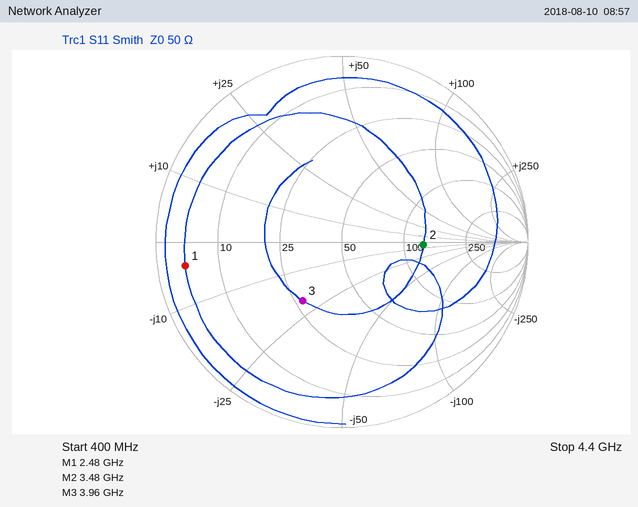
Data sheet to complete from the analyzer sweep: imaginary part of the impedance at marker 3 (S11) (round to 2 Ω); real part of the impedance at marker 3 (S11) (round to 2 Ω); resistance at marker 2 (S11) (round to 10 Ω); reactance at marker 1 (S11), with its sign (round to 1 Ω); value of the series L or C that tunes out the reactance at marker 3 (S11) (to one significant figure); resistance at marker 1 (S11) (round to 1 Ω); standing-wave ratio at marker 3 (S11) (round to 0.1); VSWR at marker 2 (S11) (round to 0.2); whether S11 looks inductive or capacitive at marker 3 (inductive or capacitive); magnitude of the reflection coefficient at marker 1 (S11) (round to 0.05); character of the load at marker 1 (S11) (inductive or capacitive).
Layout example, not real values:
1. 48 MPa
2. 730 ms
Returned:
1. -20 Ω
2. 28 Ω
3. 130 Ω
4. -4 Ω
5. 800 pH
6. 4 Ω
7. 2.2
8. 2.6
9. capacitive
10. 0.85
11. capacitive
